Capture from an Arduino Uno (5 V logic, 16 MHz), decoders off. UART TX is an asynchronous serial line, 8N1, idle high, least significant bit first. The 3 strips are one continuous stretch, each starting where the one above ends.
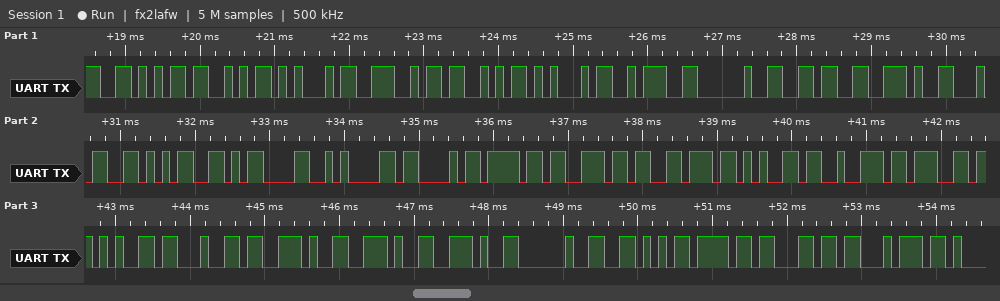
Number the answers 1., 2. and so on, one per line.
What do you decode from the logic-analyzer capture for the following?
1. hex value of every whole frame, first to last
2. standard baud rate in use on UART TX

1. 56 53 45 4E 53 45 3A 20 36 2E 34 35 0D 0A 43 6F 6E 76 65 72 67 65 64 2E 2E 2E 20 56 6F 6C 74
2. 9600 baud
